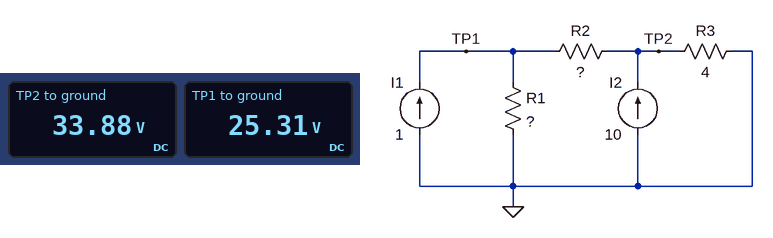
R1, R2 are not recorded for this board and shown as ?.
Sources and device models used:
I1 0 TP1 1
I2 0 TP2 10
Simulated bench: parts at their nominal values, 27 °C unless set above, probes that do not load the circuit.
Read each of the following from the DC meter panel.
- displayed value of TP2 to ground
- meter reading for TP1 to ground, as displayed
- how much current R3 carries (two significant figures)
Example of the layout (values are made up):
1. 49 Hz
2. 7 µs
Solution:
1. 33.88 V
2. 25.31 V
3. 8.5 A
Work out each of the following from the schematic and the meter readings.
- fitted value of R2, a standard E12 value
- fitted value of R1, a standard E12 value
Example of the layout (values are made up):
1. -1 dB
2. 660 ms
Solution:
1. 5.6 Ω
2. 10 Ω
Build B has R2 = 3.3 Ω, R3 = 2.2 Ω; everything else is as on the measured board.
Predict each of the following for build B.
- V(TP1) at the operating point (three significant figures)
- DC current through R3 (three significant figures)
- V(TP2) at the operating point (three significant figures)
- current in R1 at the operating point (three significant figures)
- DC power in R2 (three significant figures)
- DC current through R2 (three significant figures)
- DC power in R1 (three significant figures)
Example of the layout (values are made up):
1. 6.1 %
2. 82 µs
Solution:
1. 17.7 V
2. 9.23 A
3. 20.3 V
4. 1.77 A
5. 1.98 W
6. 774 mA
7. 31.5 W
